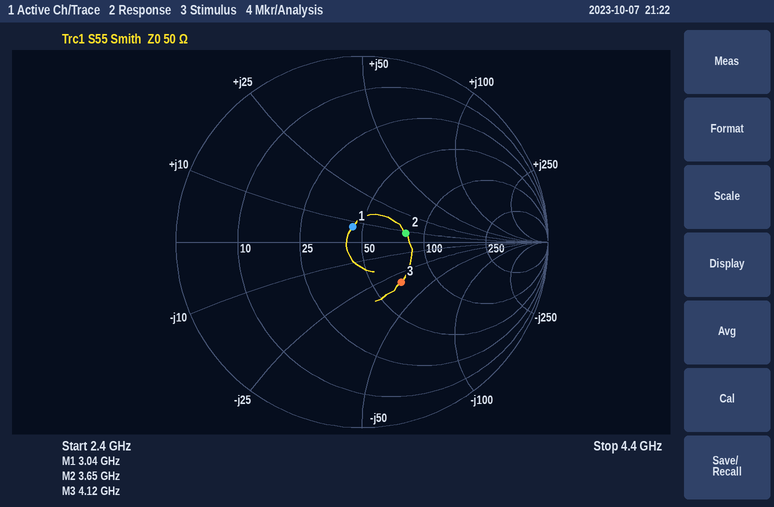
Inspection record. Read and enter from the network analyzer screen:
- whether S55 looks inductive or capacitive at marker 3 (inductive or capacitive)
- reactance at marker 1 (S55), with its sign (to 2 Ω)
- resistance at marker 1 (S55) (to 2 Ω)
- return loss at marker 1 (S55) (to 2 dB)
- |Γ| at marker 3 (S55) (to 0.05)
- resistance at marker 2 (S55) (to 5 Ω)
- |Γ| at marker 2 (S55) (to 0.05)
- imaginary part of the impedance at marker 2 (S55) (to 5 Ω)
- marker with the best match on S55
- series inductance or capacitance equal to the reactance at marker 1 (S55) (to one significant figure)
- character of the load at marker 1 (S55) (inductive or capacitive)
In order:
capacitive
+8 Ω
44 Ω
20 dB
0.30
80 Ω
0.25
+10 Ω
marker 1
400 pH
inductive
